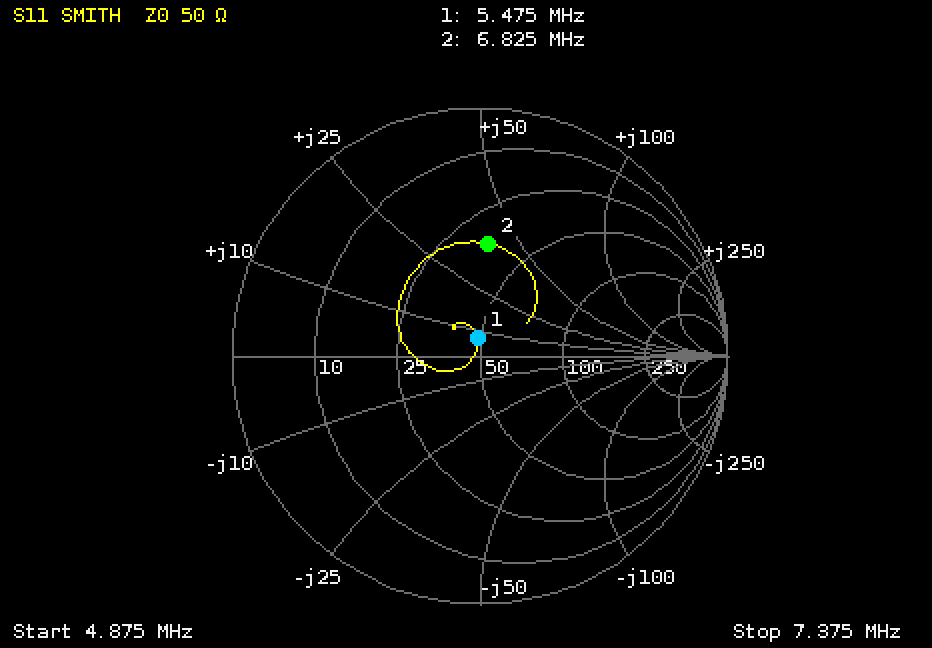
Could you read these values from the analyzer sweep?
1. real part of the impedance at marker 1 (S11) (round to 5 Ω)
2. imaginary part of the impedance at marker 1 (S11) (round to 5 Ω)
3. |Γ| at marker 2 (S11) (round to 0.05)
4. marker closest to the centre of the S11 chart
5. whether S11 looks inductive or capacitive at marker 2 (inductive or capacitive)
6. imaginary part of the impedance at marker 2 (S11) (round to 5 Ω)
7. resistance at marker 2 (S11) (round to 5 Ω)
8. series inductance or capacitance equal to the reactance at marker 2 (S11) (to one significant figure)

50 Ω
+5 Ω
0.45
marker 1
inductive
+40 Ω
35 Ω
900 nH
